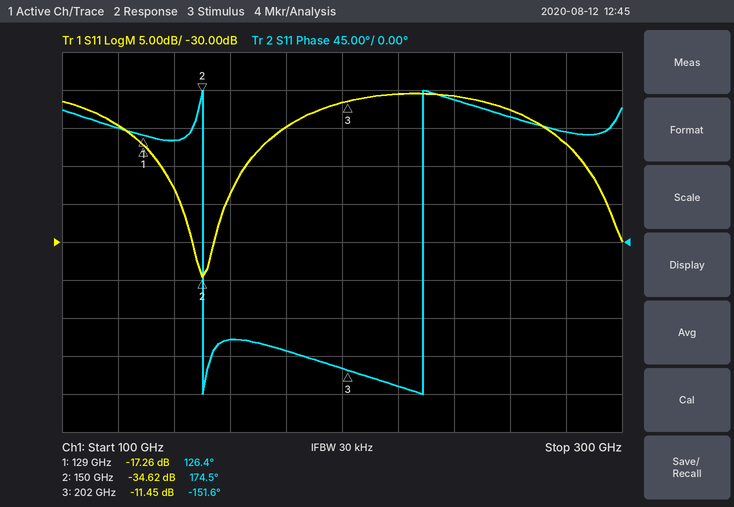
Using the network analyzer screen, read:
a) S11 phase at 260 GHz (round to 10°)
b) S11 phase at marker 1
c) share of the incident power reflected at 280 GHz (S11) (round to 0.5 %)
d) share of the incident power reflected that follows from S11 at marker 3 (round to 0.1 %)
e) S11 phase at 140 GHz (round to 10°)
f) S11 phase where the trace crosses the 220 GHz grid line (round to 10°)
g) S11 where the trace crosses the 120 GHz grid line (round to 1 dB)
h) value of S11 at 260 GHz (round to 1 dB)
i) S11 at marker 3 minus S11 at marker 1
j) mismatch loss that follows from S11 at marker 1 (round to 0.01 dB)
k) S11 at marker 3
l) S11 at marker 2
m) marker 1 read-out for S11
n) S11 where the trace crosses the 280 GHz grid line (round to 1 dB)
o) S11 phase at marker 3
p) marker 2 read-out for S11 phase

150°
126.4°
2.0 %
7.2 %
120°
-170°
-15 dB
-13 dB
5.81 dB
0.08 dB
-11.45 dB
-34.62 dB
-17.26 dB
-17 dB
-151.6°
174.5°
